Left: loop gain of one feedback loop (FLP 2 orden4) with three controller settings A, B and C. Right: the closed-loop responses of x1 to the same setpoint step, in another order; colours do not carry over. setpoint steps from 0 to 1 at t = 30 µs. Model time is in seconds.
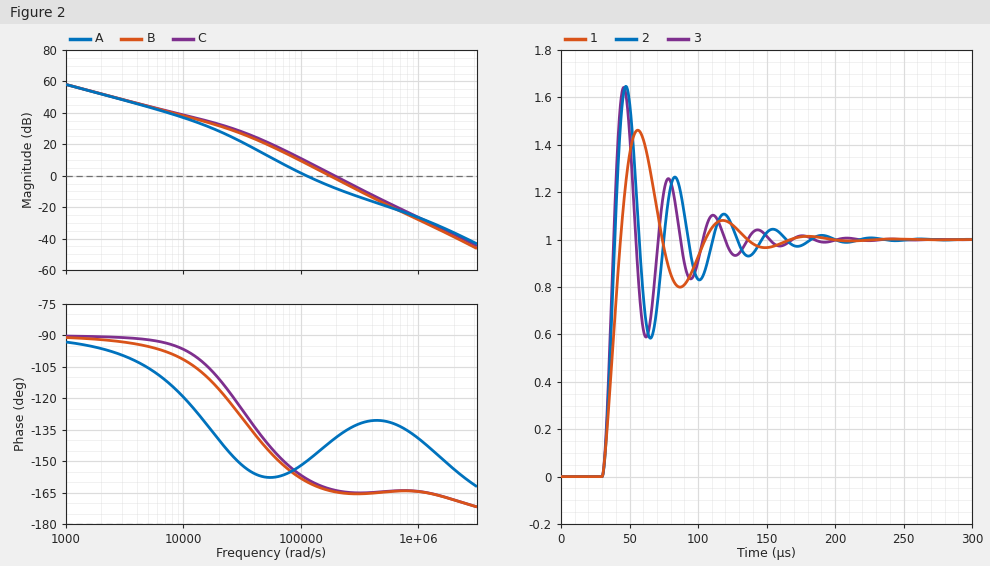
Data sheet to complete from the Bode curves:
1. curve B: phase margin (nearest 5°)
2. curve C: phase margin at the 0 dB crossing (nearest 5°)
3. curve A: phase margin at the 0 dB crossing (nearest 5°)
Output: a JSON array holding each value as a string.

["15°", "15°", "30°"]
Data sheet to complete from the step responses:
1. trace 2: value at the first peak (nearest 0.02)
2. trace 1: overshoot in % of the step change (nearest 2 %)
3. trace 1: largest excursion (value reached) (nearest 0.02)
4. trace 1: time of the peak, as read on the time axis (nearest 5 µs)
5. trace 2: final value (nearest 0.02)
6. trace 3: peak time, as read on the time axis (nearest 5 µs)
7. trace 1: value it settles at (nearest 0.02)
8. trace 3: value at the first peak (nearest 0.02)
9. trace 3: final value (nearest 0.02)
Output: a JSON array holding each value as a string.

["1.64", "46 %", "1.46", "55 µs", "1.00", "45 µs", "1.00", "1.64", "1.00"]
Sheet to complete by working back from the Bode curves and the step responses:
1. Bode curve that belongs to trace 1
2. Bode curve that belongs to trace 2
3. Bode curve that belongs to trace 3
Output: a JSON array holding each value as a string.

["A", "B", "C"]
